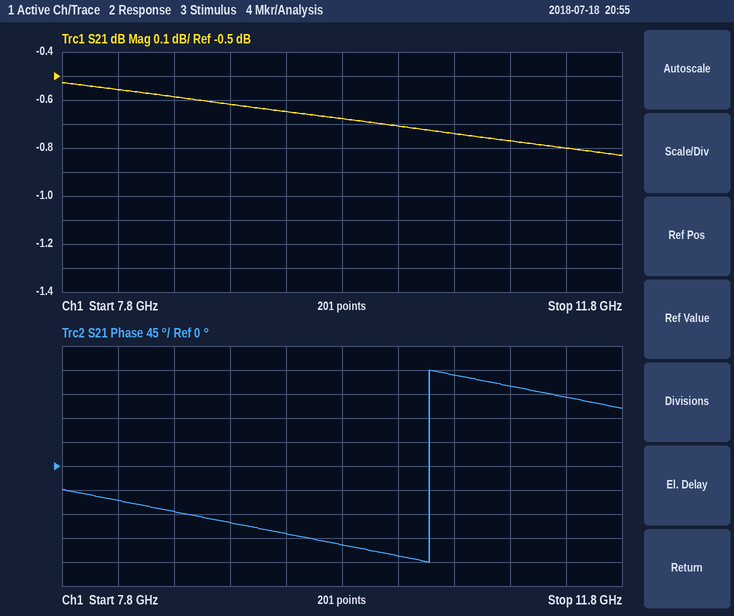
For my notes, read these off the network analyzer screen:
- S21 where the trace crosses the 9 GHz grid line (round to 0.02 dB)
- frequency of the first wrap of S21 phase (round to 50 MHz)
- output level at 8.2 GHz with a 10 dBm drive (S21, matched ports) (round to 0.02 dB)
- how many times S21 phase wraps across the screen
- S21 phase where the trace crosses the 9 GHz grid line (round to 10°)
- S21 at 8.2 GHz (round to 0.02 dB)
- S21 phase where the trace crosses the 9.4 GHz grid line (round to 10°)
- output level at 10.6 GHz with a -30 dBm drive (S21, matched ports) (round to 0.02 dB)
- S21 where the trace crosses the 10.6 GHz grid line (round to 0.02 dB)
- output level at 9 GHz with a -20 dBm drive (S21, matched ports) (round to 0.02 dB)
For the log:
-0.62 dB
10.40 GHz
9.44 dBm
1
-110°
-0.56 dB
-130°
-30.74 dBm
-0.74 dB
-20.62 dBm
